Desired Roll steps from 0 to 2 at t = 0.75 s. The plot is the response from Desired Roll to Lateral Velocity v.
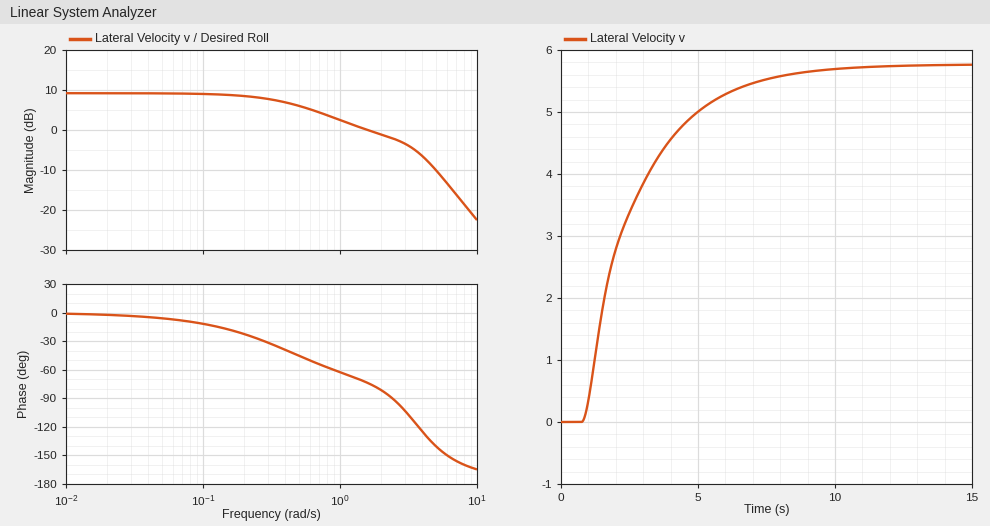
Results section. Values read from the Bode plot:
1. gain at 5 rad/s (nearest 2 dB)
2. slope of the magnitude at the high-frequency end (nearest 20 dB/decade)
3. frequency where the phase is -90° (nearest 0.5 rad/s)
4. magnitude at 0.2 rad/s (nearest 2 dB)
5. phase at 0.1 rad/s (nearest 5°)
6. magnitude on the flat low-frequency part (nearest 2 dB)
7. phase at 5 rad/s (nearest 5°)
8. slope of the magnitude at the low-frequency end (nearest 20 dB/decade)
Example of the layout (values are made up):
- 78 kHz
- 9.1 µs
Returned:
- -10 dB
- -40 dB/decade
- 2.5 rad/s
- 8 dB
- -10°
- 10 dB
- -140°
- 0 dB/decade
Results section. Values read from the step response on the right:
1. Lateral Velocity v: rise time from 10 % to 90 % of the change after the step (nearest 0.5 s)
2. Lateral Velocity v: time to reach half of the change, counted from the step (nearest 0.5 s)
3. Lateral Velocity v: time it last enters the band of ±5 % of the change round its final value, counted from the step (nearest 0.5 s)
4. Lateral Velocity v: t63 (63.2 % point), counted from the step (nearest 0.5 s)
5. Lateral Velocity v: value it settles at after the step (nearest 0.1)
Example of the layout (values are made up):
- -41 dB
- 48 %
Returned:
- 4.5 s
- 1.5 s
- 6.5 s
- 2.0 s
- 5.8
